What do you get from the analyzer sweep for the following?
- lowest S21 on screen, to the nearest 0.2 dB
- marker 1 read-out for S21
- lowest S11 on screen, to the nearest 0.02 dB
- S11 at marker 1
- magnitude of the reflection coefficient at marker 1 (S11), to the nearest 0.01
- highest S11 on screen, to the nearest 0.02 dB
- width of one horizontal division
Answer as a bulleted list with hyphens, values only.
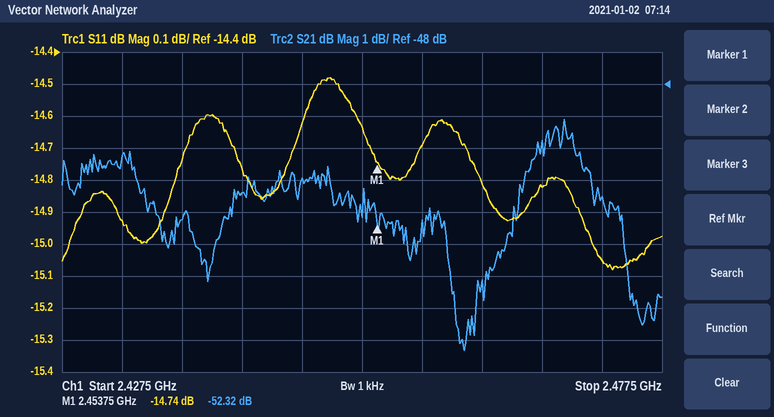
- -56.4 dB
- -52.32 dB
- -15.08 dB
- -14.74 dB
- 0.18
- -14.48 dB
- 5 MHz
